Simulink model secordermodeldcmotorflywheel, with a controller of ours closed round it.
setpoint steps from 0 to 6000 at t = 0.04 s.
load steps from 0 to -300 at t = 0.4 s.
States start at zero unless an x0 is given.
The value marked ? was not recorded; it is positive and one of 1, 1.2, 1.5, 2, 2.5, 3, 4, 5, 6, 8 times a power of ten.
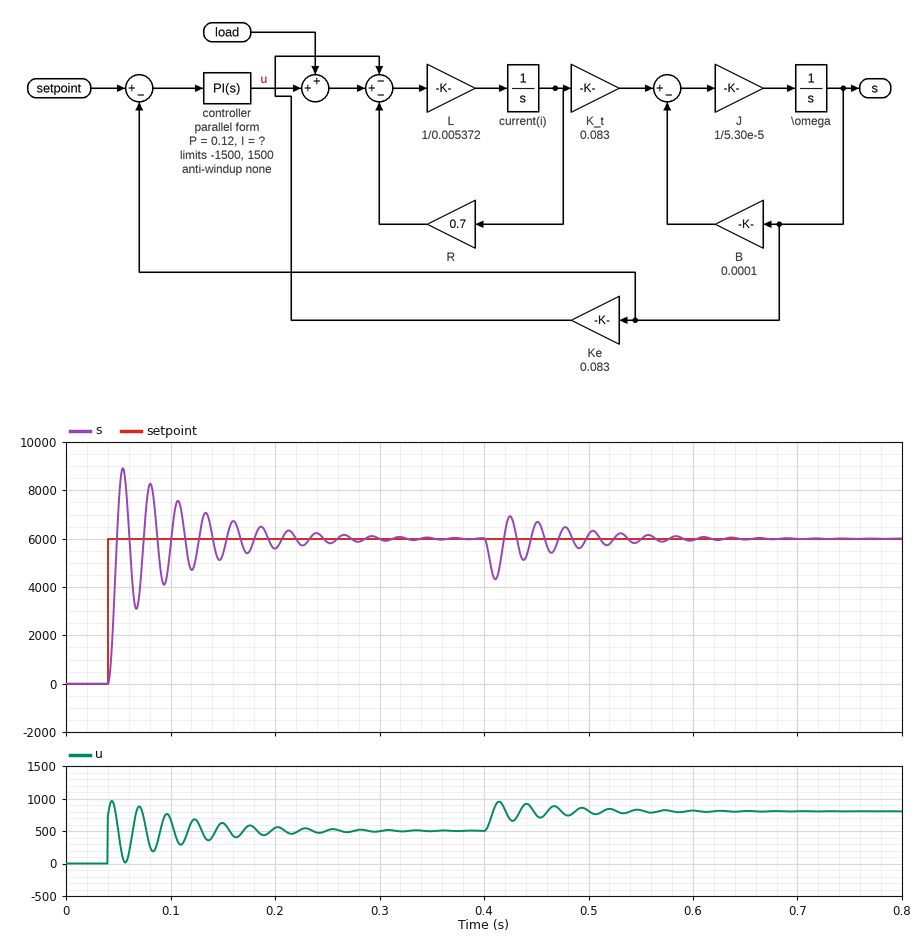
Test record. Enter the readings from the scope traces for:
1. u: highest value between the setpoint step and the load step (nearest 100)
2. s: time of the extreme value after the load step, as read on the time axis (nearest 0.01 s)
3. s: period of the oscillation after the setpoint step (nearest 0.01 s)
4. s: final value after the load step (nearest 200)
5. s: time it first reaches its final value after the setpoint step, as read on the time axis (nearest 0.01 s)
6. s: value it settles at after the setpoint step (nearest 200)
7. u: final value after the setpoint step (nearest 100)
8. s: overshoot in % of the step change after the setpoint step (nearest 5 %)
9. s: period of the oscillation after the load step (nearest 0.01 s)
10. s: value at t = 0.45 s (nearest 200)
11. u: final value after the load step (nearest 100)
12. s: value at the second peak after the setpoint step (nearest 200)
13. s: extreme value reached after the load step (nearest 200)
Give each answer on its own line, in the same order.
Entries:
1000
0.41 s
0.03 s
6000
0.05 s
6000
500
50 %
0.03 s
6600
800
8200
4400
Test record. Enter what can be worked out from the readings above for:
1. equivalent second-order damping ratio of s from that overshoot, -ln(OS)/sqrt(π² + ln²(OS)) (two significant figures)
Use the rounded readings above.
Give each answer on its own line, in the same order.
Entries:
0.22
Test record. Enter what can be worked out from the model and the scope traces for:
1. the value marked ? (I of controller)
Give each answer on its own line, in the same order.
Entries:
20
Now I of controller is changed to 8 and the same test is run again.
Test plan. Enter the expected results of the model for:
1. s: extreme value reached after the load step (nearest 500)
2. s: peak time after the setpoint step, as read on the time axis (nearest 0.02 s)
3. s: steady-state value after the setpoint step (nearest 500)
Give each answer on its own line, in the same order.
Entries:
4000
0.06 s
6000
